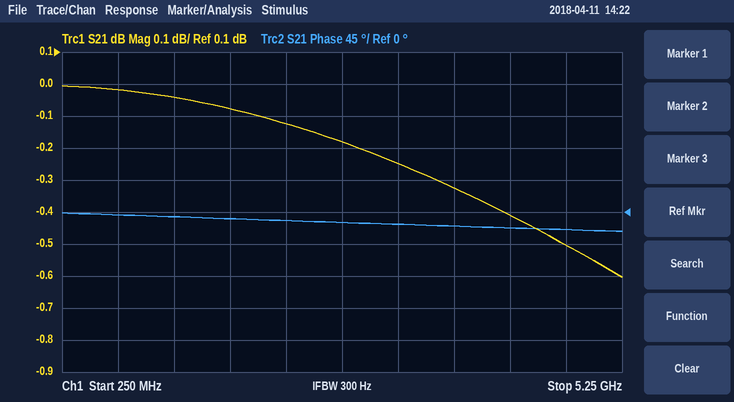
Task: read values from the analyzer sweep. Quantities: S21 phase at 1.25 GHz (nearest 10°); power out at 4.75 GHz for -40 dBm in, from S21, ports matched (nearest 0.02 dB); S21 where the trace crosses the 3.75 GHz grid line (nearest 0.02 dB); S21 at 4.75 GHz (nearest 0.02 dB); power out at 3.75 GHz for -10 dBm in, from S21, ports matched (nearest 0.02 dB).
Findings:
-10°
-40.50 dBm
-0.32 dB
-0.50 dB
-10.32 dBm
